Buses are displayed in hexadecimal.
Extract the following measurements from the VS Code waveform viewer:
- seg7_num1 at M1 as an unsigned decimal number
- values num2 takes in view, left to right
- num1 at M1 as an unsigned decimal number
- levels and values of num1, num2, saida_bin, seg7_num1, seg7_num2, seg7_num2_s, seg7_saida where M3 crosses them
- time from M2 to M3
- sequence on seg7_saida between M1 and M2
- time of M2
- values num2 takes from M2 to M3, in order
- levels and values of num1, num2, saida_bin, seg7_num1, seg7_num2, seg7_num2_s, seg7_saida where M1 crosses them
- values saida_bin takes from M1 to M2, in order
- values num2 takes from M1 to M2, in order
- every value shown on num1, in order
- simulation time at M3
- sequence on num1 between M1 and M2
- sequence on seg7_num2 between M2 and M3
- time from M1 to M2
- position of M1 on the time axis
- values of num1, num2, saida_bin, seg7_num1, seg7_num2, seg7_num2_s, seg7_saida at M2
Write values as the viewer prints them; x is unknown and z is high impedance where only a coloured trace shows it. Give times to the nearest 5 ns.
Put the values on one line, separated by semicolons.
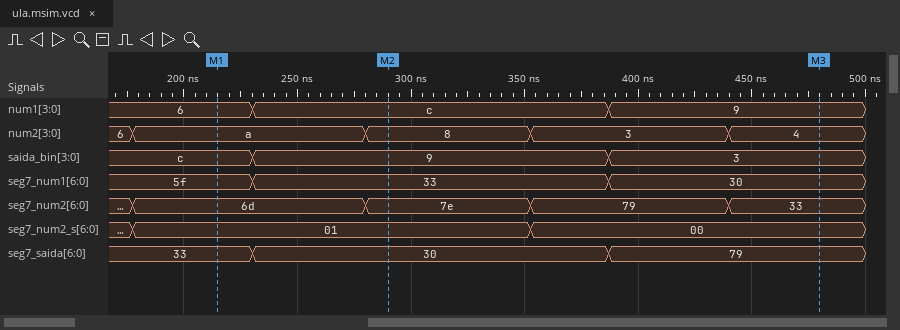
95; 6, a, 8, 3, 4; 6; num1=9, num2=4, saida_bin=3, seg7_num1=30, seg7_num2=33, seg7_num2_s=00, seg7_saida=79; 190 ns; 33, 30; 290 ns; 8, 3, 4; num1=6, num2=a, saida_bin=c, seg7_num1=5f, seg7_num2=6d, seg7_num2_s=01, seg7_saida=33; c, 9; a, 8; 6, c, 9; 480 ns; 6, c; 7e, 79, 33; 75 ns; 215 ns; num1=c, num2=8, saida_bin=9, seg7_num1=33, seg7_num2=7e, seg7_num2_s=01, seg7_saida=30
